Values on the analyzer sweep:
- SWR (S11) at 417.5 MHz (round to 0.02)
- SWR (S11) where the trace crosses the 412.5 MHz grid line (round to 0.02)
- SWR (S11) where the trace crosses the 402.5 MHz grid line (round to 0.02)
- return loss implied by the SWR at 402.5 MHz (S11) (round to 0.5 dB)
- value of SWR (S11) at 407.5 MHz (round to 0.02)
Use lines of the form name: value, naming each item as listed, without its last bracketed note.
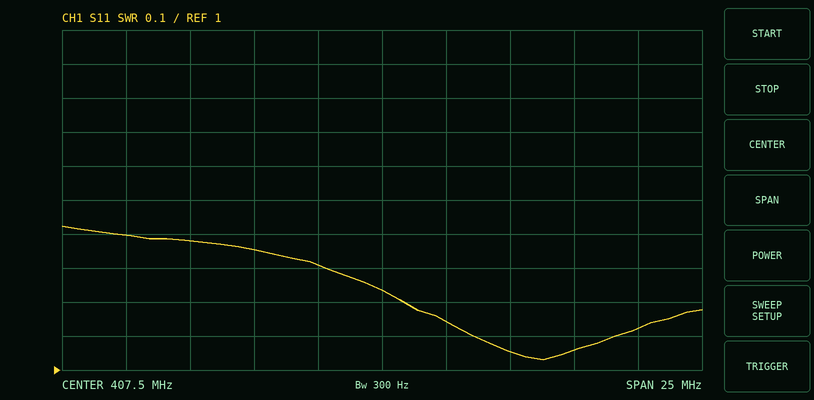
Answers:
SWR (S11) at 417.5 MHz: 1.12
SWR (S11) where the trace crosses the 412.5 MHz grid line: 1.06
SWR (S11) where the trace crosses the 402.5 MHz grid line: 1.36
return loss implied by the SWR at 402.5 MHz (S11): 16.5 dB
value of SWR (S11) at 407.5 MHz: 1.24
